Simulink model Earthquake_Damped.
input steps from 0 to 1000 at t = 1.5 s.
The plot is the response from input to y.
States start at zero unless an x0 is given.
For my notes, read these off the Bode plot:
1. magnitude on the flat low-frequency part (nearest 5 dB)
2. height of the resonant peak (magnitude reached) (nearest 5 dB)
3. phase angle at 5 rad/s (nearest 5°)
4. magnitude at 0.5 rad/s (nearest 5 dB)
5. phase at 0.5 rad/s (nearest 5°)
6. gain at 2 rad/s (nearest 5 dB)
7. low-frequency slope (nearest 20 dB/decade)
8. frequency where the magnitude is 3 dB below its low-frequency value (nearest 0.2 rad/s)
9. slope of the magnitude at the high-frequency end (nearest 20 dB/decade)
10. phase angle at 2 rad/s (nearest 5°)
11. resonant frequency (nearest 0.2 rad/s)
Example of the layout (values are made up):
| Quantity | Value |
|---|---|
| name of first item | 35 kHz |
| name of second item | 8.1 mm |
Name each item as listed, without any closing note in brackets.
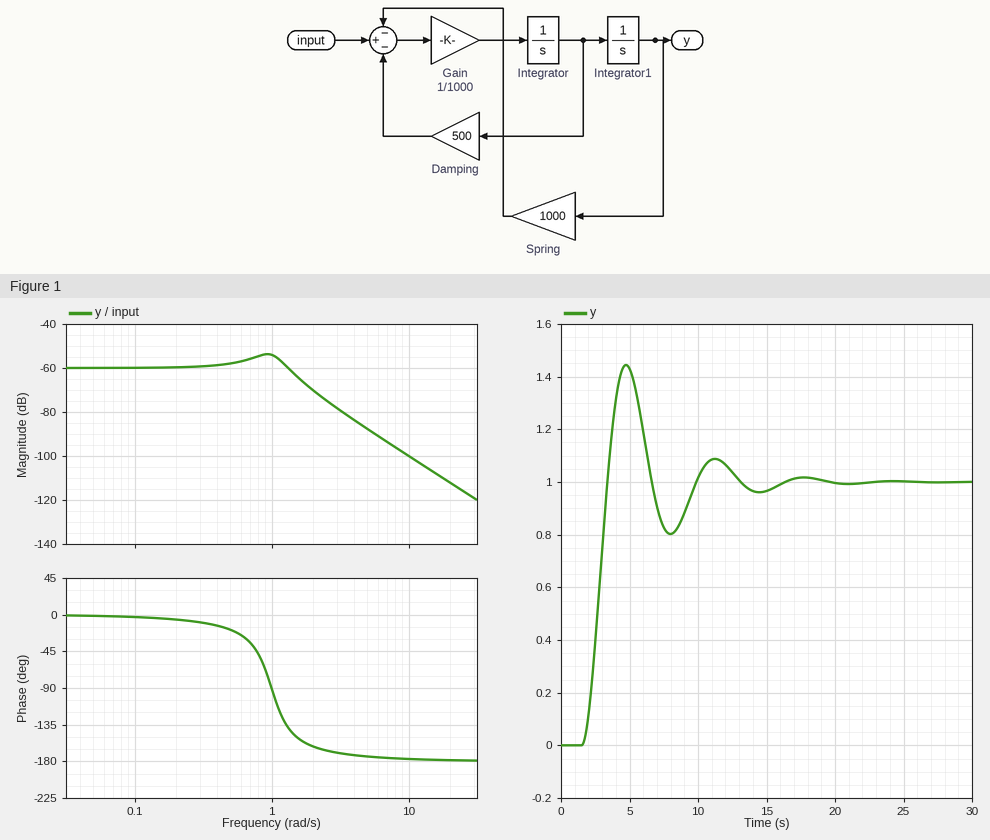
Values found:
| Quantity | Value |
|---|---|
| magnitude on the flat low-frequency part | -60 dB |
| height of the resonant peak (magnitude reached) | -55 dB |
| phase angle at 5 rad/s | -175° |
| magnitude at 0.5 rad/s | -60 dB |
| phase at 0.5 rad/s | -20° |
| gain at 2 rad/s | -70 dB |
| low-frequency slope | 0 dB/decade |
| frequency where the magnitude is 3 dB below its low-frequency value | 1.4 rad/s |
| slope of the magnitude at the high-frequency end | -40 dB/decade |
| phase angle at 2 rad/s | -160° |
| resonant frequency | 1.0 rad/s |
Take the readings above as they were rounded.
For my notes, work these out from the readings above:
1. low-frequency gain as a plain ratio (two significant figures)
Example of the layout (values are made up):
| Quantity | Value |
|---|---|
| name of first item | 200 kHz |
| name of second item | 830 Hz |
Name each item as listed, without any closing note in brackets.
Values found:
| Quantity | Value |
|---|---|
| low-frequency gain as a plain ratio | 0.0010 |
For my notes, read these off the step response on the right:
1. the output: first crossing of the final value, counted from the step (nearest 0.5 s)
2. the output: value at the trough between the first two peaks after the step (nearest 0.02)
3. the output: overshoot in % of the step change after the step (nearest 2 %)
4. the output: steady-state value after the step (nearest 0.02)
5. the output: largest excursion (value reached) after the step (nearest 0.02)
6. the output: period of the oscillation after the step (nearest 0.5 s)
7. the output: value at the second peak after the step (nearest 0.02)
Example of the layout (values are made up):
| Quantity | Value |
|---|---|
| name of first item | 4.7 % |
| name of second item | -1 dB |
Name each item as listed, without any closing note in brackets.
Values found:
| Quantity | Value |
|---|---|
| the output: first crossing of the final value, counted from the step | 2.0 s |
| the output: value at the trough between the first two peaks after the step | 0.80 |
| the output: overshoot in % of the step change after the step | 44 % |
| the output: steady-state value after the step | 1.00 |
| the output: largest excursion (value reached) after the step | 1.44 |
| the output: period of the oscillation after the step | 6.5 s |
| the output: value at the second peak after the step | 1.08 |
